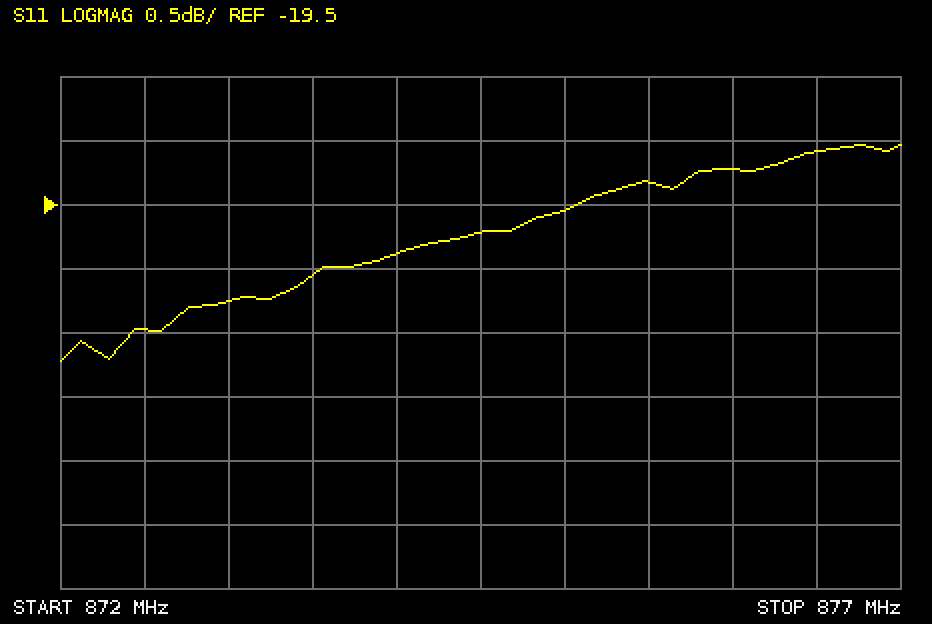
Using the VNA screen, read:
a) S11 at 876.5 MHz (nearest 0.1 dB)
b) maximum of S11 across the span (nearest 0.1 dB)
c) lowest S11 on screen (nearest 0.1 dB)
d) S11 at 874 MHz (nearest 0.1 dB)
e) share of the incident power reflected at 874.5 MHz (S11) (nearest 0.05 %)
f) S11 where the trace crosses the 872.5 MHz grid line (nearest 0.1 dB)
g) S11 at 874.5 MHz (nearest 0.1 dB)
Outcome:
-19.1 dB
-19.0 dB
-20.7 dB
-19.9 dB
1.05 %
-20.5 dB
-19.7 dB
